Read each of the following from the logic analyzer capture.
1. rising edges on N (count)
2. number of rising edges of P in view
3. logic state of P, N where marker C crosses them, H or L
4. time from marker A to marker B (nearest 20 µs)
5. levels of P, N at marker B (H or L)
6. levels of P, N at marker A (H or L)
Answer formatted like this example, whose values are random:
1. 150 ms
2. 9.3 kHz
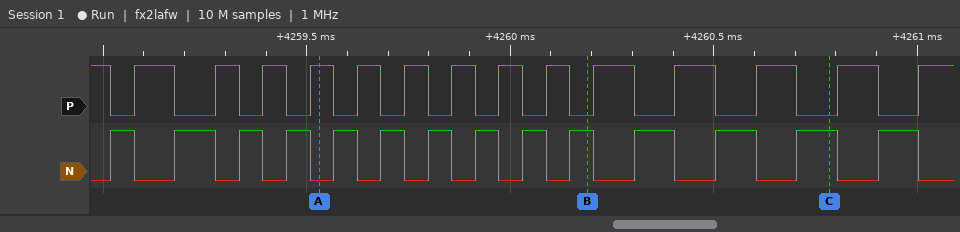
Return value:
1. 14
2. 14
3. P=L, N=H
4. 660 µs
5. P=L, N=H
6. P=H, N=L
